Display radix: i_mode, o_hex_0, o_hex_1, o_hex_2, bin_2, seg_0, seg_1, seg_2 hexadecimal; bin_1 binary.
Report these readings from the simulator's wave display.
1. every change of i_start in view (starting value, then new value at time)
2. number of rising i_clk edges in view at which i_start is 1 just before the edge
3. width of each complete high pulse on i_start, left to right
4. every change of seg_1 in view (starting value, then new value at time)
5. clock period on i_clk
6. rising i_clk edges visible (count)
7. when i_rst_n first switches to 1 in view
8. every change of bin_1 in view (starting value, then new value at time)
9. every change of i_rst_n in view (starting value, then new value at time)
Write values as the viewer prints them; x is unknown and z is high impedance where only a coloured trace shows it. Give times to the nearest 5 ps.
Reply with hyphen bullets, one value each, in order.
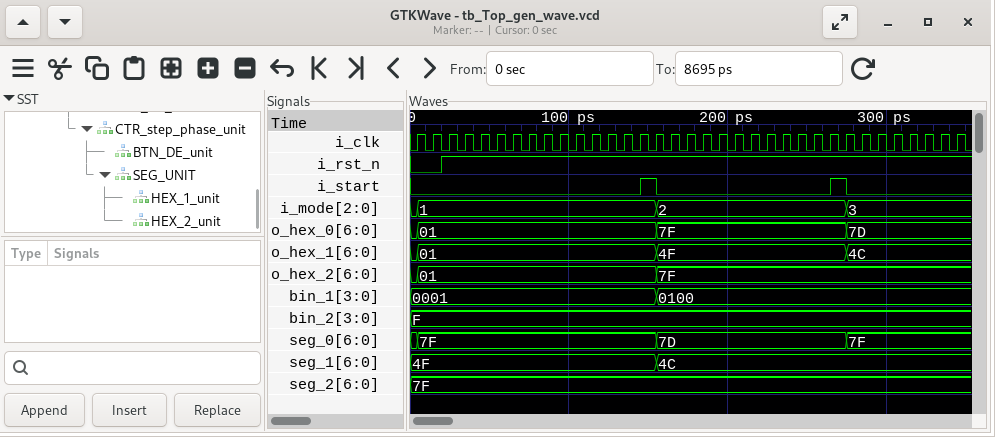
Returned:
- 0, 1 at 145 ps, 0 at 155 ps, 1 at 265 ps, 0 at 275 ps
- 2
- 10 ps, 10 ps
- 4F, 4C at 155 ps
- 10 ps
- 35
- 20 ps
- 0001, 0100 at 155 ps
- 0, 1 at 20 ps
